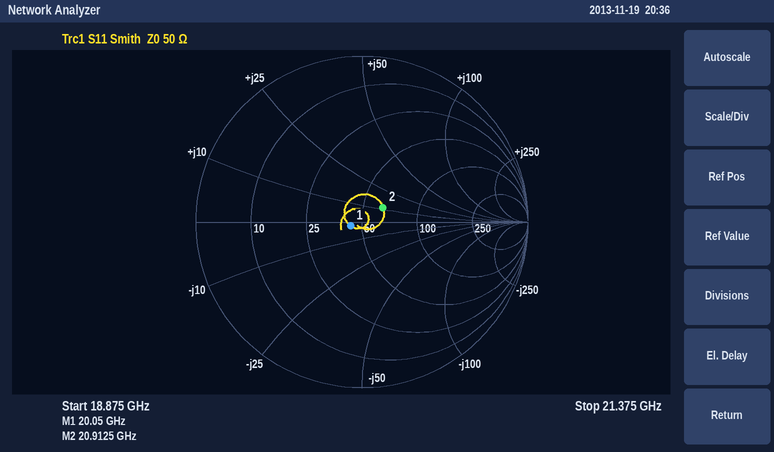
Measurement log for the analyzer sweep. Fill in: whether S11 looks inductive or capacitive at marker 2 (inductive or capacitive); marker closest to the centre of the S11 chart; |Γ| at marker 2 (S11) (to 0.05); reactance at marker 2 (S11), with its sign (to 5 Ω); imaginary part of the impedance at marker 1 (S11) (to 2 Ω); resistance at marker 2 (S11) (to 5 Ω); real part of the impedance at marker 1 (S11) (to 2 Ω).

inductive
marker 1
0.15
+10 Ω
-2 Ω
65 Ω
44 Ω
